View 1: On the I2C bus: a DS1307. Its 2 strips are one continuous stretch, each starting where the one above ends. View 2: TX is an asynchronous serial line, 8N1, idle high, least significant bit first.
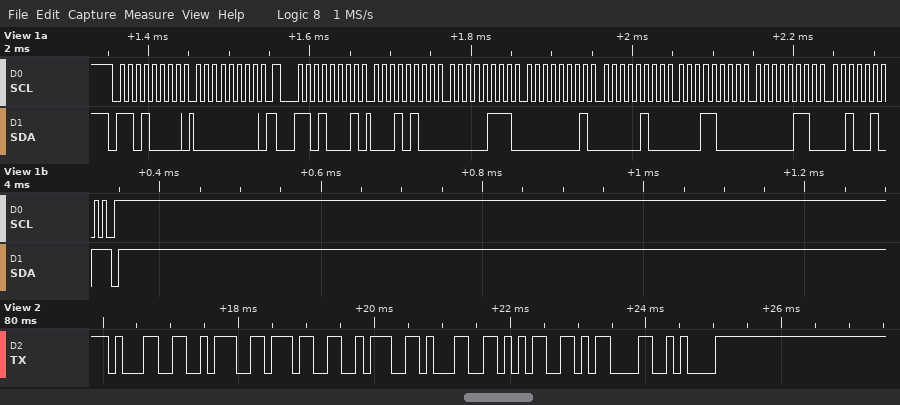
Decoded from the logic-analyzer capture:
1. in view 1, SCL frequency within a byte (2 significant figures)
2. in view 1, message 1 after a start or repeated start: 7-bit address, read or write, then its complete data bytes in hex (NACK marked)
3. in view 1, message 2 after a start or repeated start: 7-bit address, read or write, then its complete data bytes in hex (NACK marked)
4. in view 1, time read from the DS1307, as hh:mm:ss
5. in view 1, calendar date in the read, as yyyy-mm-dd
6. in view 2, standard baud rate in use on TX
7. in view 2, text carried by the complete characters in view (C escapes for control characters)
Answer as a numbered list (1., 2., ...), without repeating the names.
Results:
1. 100 kHz
2. 0x68 write: 00
3. 0x68 read: 14 07 01 04 18 06 25 NACK
4. 01:07:14
5. 2025-06-18
6. 9600 baud
7. "1:7:15\r\n"
